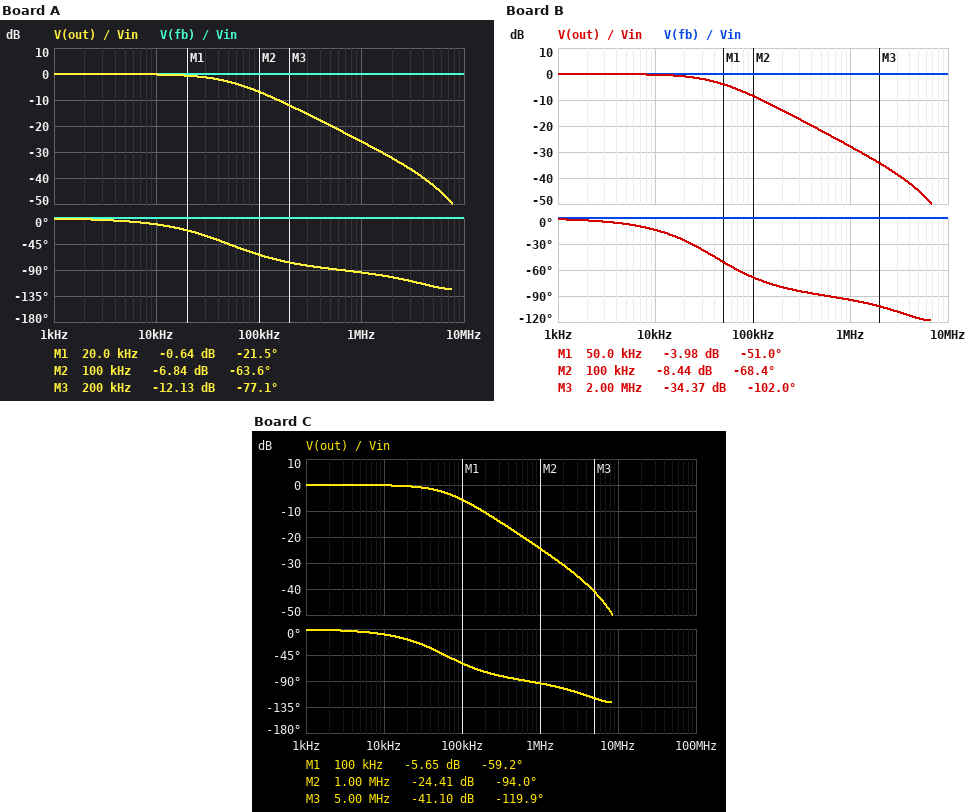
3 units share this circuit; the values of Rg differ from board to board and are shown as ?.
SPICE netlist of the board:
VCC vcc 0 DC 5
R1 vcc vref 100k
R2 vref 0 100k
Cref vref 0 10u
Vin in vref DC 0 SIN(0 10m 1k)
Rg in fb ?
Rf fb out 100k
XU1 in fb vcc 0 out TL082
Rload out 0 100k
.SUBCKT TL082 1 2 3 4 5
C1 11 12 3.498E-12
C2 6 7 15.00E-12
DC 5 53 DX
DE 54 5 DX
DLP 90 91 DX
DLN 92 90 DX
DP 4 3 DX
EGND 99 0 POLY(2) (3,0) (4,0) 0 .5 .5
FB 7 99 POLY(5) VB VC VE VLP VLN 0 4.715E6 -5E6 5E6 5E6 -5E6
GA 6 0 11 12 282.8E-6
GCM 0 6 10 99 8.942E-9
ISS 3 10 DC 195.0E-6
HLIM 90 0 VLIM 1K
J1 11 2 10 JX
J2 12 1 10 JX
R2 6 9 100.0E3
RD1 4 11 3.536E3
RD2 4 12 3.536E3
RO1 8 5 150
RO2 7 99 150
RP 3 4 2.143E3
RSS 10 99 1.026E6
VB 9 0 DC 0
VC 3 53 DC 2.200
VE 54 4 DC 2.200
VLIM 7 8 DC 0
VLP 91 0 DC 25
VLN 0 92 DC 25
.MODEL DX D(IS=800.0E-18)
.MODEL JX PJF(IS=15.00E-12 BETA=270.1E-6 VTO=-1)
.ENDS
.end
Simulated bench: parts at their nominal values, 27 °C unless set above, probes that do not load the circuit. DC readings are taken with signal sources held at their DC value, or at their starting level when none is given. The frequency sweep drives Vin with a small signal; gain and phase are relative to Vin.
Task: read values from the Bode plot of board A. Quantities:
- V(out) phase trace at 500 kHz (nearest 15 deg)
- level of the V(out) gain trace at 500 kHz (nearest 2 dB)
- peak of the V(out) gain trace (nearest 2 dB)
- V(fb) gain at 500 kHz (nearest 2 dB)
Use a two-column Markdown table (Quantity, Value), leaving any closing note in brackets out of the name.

| Quantity | Value |
|---|---|
| V(out) phase trace at 500 kHz | -90 deg |
| level of the V(out) gain trace at 500 kHz | -20 dB |
| peak of the V(out) gain trace | 0 dB |
| V(fb) gain at 500 kHz | 0 dB |
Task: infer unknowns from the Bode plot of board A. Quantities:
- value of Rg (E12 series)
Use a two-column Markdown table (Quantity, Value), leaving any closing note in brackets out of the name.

| Quantity | Value |
|---|---|
| value of Rg | 1.5 kΩ |
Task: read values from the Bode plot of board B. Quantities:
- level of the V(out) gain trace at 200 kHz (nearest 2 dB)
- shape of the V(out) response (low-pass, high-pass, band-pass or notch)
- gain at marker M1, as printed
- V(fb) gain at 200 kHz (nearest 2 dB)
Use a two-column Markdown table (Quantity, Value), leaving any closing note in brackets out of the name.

| Quantity | Value |
|---|---|
| level of the V(out) gain trace at 200 kHz | -14 dB |
| shape of the V(out) response | low-pass |
| gain at marker M1, as printed | -3.98 dB |
| V(fb) gain at 200 kHz | 0 dB |
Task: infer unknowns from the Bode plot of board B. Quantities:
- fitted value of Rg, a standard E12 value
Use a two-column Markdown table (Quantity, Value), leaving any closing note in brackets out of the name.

| Quantity | Value |
|---|---|
| fitted value of Rg, a standard E12 value | 1.2 kΩ |
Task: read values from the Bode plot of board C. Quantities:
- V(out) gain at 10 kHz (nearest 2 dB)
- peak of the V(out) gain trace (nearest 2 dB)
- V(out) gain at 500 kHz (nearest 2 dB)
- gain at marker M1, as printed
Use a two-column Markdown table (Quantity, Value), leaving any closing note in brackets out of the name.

| Quantity | Value |
|---|---|
| V(out) gain at 10 kHz | 0 dB |
| peak of the V(out) gain trace | 0 dB |
| V(out) gain at 500 kHz | -18 dB |
| gain at marker M1, as printed | -5.65 dB |
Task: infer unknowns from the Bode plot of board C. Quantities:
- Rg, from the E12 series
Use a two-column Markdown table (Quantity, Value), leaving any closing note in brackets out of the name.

| Quantity | Value |
|---|---|
| Rg, from the E12 series | 1.8 kΩ |
